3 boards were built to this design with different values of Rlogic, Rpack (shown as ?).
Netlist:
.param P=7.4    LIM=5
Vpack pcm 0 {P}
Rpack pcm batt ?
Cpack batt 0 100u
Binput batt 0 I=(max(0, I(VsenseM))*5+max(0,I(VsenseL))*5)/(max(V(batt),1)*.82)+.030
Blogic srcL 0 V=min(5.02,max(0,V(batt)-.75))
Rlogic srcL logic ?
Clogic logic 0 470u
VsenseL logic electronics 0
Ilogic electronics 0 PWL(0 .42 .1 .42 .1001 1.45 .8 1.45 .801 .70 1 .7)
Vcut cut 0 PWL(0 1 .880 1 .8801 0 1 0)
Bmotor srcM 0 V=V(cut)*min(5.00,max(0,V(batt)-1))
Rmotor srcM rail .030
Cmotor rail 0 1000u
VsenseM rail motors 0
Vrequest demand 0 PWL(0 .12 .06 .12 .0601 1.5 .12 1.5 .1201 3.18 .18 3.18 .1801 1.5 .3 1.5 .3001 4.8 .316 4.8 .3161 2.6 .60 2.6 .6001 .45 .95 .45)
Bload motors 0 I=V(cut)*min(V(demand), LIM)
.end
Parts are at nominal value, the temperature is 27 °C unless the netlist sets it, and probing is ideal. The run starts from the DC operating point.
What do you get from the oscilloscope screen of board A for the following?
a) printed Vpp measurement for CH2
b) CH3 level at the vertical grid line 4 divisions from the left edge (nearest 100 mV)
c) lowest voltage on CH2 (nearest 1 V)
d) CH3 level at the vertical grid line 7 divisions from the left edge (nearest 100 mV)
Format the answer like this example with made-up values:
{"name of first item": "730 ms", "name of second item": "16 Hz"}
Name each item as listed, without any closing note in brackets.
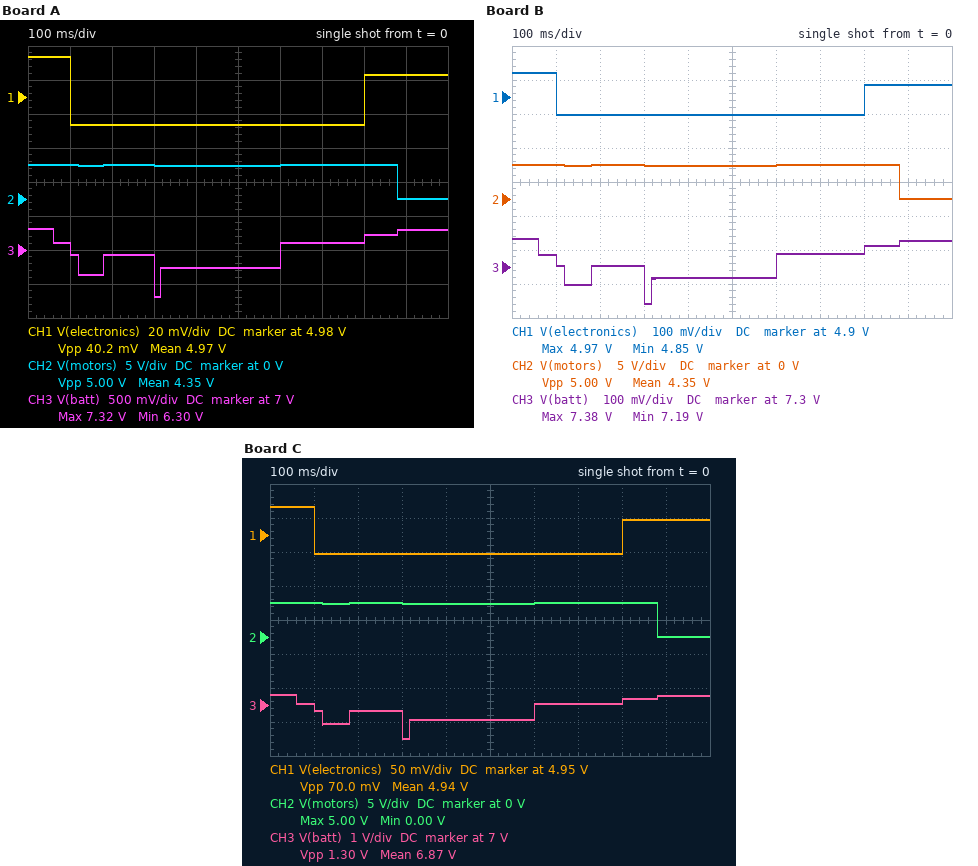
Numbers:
{"printed Vpp measurement for CH2": "5.00 V", "CH3 level at the vertical grid line 4 divisions from the left edge": "6.7 V", "lowest voltage on CH2": "0 V", "CH3 level at the vertical grid line 7 divisions from the left edge": "7.1 V"}
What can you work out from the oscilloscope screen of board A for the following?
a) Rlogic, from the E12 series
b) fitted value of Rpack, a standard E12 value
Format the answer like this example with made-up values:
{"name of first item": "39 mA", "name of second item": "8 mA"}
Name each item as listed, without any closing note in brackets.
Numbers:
{"Rlogic, from the E12 series": "0.039 Ω", "fitted value of Rpack, a standard E12 value": "0.18 Ω"}
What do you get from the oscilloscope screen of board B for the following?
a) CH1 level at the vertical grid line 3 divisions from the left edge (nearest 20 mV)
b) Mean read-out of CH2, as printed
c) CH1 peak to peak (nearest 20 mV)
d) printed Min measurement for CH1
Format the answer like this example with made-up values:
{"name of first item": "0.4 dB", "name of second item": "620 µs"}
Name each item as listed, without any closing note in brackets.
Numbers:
{"CH1 level at the vertical grid line 3 divisions from the left edge": "4.84 V", "Mean read-out of CH2, as printed": "4.35 V", "CH1 peak to peak": "120 mV", "printed Min measurement for CH1": "4.85 V"}
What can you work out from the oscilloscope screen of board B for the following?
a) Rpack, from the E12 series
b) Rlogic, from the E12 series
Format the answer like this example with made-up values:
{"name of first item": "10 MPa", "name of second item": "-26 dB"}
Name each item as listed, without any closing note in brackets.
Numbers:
{"Rpack, from the E12 series": "0.039 Ω", "Rlogic, from the E12 series": "0.12 Ω"}
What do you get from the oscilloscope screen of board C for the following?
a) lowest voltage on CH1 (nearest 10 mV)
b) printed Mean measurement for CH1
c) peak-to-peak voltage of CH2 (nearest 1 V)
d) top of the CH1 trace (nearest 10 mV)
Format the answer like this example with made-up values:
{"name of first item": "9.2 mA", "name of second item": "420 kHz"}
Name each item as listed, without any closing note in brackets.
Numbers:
{"lowest voltage on CH1": "4.92 V", "printed Mean measurement for CH1": "4.94 V", "peak-to-peak voltage of CH2": "5 V", "top of the CH1 trace": "4.99 V"}
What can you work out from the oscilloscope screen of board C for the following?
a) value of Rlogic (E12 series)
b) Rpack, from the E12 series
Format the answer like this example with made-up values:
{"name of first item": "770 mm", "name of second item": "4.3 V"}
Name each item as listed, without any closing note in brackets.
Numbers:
{"value of Rlogic": "0.068 Ω", "Rpack, from the E12 series": "0.22 Ω"}
